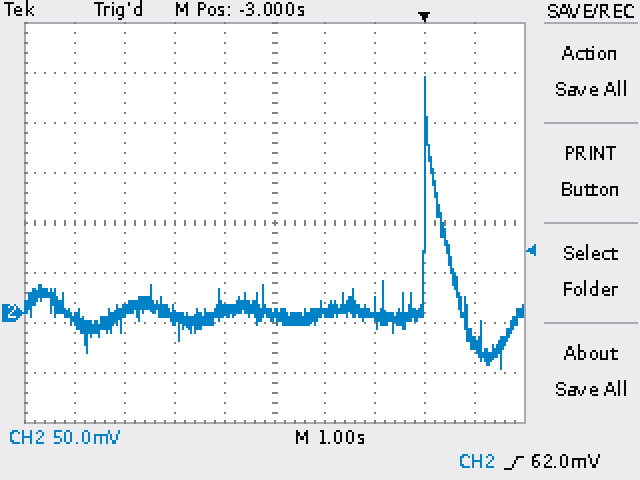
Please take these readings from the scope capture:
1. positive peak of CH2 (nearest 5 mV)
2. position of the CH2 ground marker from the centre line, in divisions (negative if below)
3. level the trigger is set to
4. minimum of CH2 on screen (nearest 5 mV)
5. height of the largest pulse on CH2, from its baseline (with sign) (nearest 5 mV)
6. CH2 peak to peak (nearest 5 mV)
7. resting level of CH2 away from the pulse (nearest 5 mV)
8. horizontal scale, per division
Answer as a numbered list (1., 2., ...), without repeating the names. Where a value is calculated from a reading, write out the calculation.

1. 235 mV
2. -1.8 div
3. 62.0 mV
4. -55 mV
5. 235 mV − (0 mV) = +235 mV
6. 235 mV − (-55 mV) = 290 mV
7. 0 mV
8. 1 s
